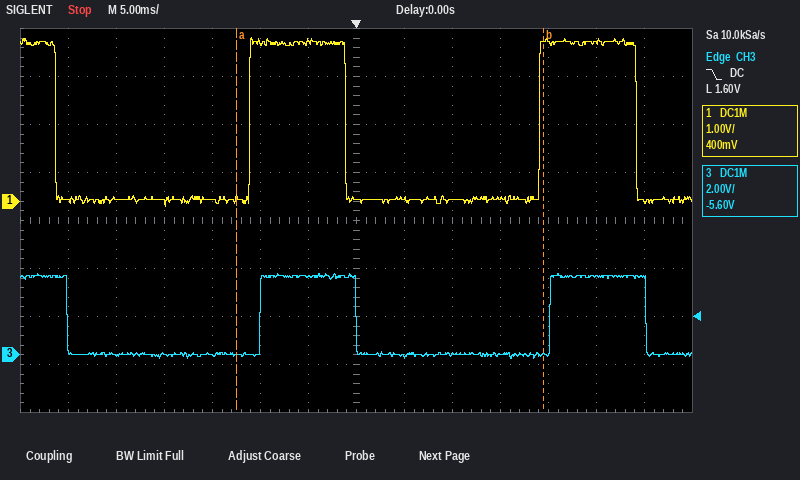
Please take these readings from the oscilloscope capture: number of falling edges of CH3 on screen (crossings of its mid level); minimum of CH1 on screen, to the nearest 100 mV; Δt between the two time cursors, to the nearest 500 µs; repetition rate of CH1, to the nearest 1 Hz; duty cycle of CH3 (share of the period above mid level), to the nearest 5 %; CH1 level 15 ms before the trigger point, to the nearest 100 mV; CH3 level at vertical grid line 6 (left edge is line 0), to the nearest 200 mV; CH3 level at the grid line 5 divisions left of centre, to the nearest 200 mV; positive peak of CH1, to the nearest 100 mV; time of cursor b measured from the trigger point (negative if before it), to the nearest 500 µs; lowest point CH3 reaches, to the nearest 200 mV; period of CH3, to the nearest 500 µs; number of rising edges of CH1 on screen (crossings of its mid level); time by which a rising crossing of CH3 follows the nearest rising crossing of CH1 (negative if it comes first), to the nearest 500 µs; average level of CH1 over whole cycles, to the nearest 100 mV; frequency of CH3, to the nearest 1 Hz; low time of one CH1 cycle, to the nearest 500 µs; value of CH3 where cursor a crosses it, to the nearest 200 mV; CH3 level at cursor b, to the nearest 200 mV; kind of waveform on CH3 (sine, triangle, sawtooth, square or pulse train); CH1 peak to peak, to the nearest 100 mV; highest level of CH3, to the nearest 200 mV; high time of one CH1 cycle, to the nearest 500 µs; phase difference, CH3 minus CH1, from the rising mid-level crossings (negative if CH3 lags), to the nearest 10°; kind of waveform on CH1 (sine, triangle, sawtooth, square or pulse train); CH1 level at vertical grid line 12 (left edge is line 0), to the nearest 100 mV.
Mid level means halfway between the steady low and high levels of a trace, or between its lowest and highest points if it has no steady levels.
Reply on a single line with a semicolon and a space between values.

3; -100 mV; 32.0 ms; 33 Hz; 35 %; 0.0 V; 3.2 V; 0.0 V; 3.4 V; +19.5 ms; -200 mV; 30.0 ms; 2; +1.0 ms; 1.1 V; 33 Hz; 20.0 ms; 0.0 V; 0.0 V; pulse train; 3.5 V; 3.4 V; 10.0 ms; -10°; pulse train; 3.3 V
